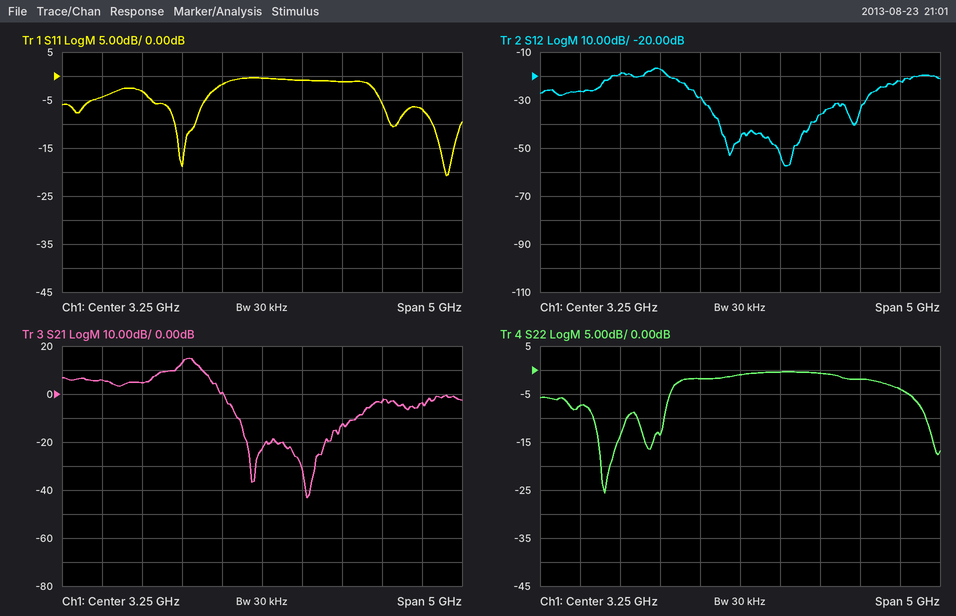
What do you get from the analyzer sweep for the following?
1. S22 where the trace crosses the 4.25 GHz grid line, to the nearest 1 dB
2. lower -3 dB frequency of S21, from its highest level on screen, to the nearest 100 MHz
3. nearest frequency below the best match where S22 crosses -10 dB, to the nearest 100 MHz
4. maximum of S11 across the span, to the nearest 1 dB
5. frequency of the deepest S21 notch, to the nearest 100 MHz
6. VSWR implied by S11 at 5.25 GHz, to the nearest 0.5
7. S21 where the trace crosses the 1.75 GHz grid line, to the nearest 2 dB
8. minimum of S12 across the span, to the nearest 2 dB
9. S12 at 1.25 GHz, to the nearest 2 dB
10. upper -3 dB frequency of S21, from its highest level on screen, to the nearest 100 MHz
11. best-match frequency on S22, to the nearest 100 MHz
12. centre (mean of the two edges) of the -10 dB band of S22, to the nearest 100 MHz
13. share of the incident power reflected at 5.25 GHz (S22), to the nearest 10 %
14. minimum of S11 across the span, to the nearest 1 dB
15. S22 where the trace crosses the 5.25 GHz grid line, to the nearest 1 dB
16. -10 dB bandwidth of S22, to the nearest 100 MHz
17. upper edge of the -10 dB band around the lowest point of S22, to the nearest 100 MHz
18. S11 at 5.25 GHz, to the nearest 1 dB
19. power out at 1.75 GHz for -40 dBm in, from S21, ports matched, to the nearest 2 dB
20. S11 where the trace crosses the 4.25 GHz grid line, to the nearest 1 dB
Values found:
-1 dB
2.2 GHz
1.4 GHz
0 dB
3.8 GHz
2.5
4 dB
-58 dB
-26 dB
2.5 GHz
1.6 GHz
1.6 GHz
40 %
-21 dB
-4 dB
400 MHz
1.8 GHz
-7 dB
-36 dBm
-1 dB
